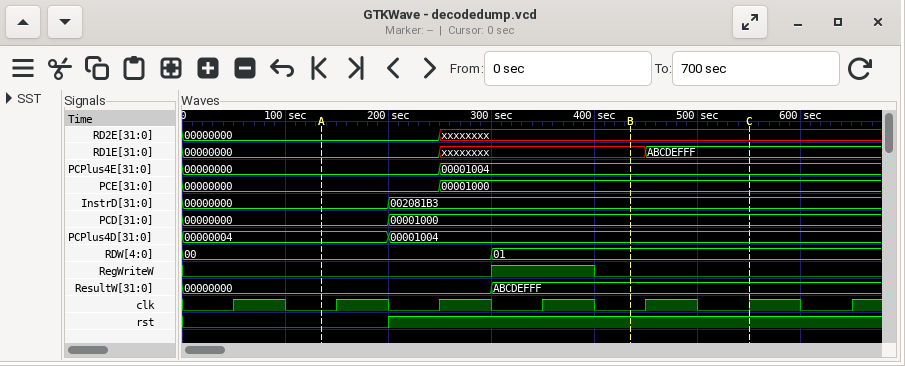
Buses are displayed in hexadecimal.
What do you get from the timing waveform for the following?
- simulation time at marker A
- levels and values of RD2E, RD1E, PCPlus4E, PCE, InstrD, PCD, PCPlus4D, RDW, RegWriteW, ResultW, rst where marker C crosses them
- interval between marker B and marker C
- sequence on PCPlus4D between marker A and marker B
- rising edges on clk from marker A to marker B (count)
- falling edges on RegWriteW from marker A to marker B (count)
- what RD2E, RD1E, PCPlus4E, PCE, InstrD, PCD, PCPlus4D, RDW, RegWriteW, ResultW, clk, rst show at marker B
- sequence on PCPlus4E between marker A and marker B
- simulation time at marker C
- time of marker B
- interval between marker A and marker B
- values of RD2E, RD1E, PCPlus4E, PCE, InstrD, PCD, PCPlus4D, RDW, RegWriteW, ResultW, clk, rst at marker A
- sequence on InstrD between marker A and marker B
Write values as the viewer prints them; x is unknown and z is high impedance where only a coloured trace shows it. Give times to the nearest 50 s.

150 s
RD2E=xxxxxxxx, RD1E=ABCDEFFF, PCPlus4E=00001004, PCE=00001000, InstrD=002081B3, PCD=00001000, PCPlus4D=00001004, RDW=01, RegWriteW=0, ResultW=ABCDEFFF, rst=1
100 s
00000004, 00001004
3
1
RD2E=xxxxxxxx, RD1E=xxxxxxxx, PCPlus4E=00001004, PCE=00001000, InstrD=002081B3, PCD=00001000, PCPlus4D=00001004, RDW=01, RegWriteW=0, ResultW=ABCDEFFF, clk=0, rst=1
00000000, 00001004
550 s
450 s
300 s
RD2E=00000000, RD1E=00000000, PCPlus4E=00000000, PCE=00000000, InstrD=00000000, PCD=00000000, PCPlus4D=00000004, RDW=00, RegWriteW=0, ResultW=00000000, clk=0, rst=0
00000000, 002081B3
